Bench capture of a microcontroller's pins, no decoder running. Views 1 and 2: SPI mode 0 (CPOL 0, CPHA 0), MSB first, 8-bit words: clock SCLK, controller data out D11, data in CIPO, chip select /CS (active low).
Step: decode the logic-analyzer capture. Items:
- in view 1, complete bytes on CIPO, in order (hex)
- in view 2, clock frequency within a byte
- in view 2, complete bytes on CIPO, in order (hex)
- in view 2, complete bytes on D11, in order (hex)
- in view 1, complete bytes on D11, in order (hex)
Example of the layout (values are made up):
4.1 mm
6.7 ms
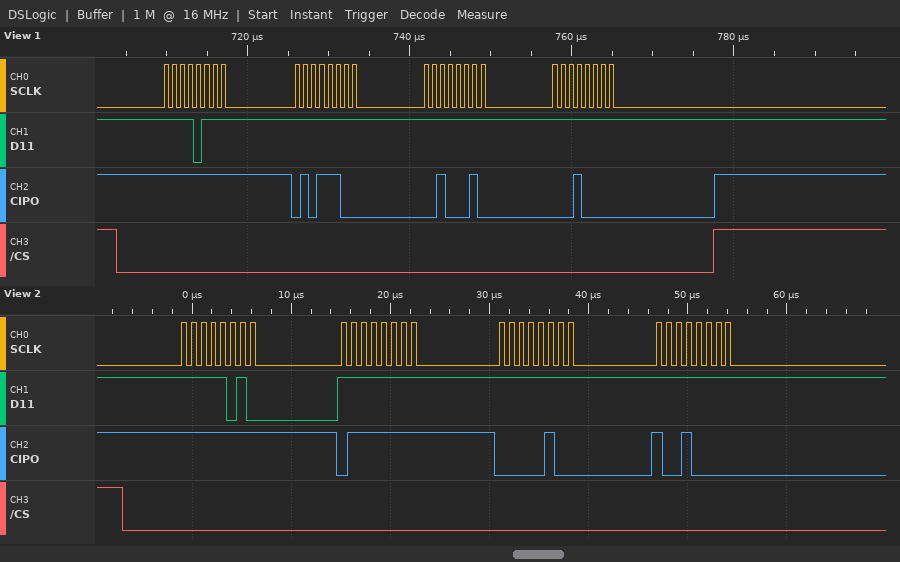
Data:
0xFF 0x5C 0x22 0x10
1 MHz
FF 7F 04 90
FA FF FF FF
0xF7 0xFF 0xFF 0xFF
